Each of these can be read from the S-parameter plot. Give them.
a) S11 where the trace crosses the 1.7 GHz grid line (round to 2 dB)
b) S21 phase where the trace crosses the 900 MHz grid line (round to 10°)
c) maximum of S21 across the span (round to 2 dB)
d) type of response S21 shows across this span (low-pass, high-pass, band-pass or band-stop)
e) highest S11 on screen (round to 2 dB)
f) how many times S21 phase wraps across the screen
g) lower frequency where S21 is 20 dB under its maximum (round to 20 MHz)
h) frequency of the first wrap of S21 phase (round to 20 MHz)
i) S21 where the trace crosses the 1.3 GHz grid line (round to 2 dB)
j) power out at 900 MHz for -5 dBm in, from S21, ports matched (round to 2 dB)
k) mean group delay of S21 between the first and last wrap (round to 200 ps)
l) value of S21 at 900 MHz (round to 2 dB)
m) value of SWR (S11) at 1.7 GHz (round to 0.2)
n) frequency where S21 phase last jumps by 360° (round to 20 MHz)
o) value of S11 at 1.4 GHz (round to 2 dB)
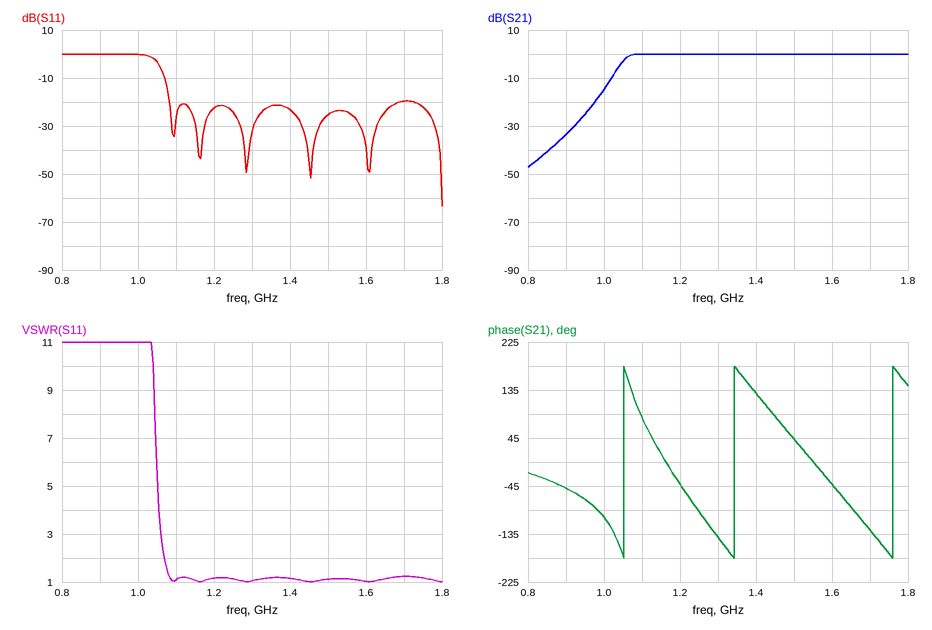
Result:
-20 dB
-50°
0 dB
high-pass
0 dB
3
980 MHz
1.06 GHz
0 dB
-38 dBm
2.8 ns
-34 dB
1.2
1.76 GHz
-24 dB
